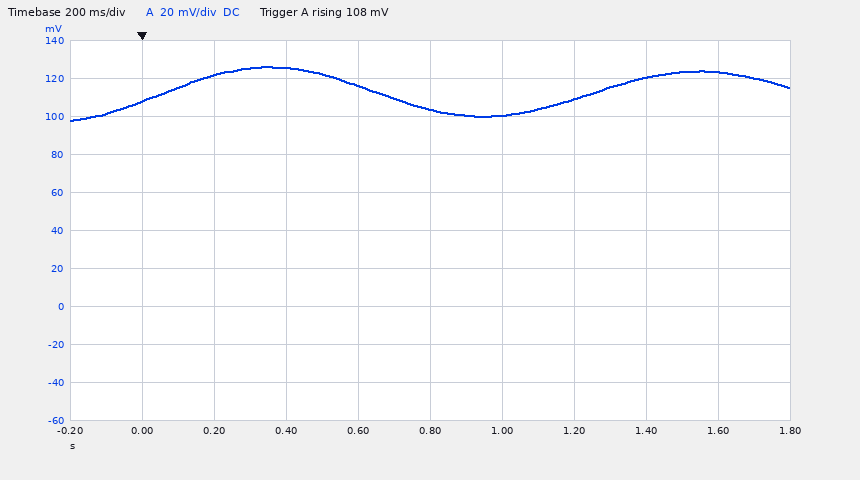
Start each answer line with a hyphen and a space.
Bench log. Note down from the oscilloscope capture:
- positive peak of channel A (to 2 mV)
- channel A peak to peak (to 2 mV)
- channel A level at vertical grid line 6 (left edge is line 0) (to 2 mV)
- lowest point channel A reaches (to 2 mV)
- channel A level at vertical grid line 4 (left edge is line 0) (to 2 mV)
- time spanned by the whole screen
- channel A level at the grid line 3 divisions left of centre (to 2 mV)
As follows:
- 126 mV
- 28 mV
- 100 mV
- 98 mV
- 116 mV
- 2 s
- 122 mV
